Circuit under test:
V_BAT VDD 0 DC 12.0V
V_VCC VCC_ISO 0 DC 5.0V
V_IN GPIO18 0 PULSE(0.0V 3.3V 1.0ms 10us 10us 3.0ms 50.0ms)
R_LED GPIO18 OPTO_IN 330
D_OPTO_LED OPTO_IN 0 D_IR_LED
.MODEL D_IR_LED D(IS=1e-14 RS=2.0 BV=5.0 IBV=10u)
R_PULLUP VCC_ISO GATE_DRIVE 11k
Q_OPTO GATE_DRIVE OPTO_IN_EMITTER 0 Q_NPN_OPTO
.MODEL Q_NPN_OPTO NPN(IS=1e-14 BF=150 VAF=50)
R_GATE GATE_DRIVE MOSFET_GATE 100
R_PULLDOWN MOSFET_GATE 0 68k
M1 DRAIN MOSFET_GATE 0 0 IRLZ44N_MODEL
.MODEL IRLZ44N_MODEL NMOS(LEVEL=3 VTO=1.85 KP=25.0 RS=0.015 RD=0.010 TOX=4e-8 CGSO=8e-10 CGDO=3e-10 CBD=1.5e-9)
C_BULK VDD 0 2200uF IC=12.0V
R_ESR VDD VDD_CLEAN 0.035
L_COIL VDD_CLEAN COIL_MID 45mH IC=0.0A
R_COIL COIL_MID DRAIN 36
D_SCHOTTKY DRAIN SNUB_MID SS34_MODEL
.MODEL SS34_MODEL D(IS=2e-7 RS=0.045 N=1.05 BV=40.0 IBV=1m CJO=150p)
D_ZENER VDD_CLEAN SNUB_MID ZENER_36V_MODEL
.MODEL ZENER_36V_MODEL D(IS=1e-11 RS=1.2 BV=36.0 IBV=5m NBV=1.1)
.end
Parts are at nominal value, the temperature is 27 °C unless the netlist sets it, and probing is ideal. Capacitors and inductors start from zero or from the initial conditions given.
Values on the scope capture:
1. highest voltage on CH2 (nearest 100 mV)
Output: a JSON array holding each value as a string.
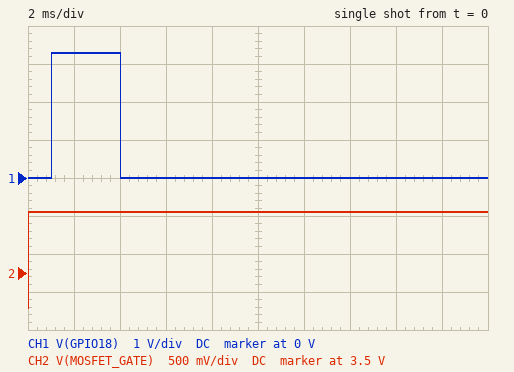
["4.3 V"]
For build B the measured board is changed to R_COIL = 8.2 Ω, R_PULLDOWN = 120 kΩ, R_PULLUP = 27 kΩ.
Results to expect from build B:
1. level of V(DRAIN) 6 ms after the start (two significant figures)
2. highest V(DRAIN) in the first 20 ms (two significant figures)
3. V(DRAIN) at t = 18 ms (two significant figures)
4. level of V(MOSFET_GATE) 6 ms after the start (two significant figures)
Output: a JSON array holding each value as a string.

["42 mV", "61 mV", "60 mV", "4.1 V"]
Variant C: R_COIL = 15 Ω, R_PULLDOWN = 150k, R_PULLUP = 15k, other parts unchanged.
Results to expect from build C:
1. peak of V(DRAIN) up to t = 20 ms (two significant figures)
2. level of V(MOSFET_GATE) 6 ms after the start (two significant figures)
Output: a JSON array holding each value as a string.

["32 mV", "4.5 V"]
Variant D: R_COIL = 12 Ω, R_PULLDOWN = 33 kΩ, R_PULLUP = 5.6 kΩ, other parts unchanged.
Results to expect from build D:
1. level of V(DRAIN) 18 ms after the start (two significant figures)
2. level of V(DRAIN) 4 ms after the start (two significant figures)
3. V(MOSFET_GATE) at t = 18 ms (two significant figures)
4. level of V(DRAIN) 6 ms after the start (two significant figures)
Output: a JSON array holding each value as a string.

["41 mV", "27 mV", "4.3 V", "33 mV"]
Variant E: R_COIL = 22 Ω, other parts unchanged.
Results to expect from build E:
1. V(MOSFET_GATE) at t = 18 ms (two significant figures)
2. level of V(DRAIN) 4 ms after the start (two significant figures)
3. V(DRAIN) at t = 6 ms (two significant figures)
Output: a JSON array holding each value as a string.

["4.3 V", "19 mV", "21 mV"]
